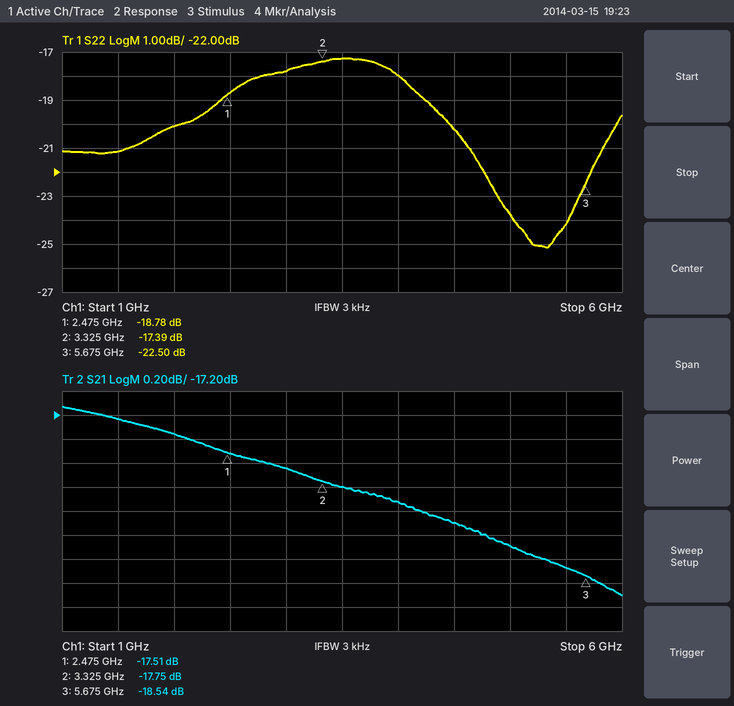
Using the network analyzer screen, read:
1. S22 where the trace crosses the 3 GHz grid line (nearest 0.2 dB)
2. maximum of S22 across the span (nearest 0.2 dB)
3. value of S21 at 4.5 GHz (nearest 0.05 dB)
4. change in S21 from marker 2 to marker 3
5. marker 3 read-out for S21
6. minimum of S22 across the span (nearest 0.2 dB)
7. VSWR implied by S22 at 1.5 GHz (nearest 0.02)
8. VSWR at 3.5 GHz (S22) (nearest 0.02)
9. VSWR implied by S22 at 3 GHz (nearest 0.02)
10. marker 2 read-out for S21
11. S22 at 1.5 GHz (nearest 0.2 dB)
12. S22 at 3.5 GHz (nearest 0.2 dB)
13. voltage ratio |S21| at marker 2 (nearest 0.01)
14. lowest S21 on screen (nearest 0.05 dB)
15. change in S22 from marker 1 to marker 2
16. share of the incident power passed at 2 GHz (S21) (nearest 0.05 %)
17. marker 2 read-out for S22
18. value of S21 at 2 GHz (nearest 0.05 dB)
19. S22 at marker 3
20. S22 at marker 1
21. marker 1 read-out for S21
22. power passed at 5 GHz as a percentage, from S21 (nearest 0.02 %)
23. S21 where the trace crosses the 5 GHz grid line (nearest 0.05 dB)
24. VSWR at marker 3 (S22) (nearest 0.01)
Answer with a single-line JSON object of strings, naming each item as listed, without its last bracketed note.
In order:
{"S22 where the trace crosses the 3 GHz grid line": "-17.8 dB", "maximum of S22 across the span": "-17.2 dB", "value of S21 at 4.5 GHz": "-18.10 dB", "change in S21 from marker 2 to marker 3": "-0.79 dB", "marker 3 read-out for S21": "-18.54 dB", "minimum of S22 across the span": "-25.2 dB", "VSWR implied by S22 at 1.5 GHz": "1.20", "VSWR at 3.5 GHz (S22)": "1.32", "VSWR implied by S22 at 3 GHz": "1.30", "marker 2 read-out for S21": "-17.75 dB", "S22 at 1.5 GHz": "-21.2 dB", "S22 at 3.5 GHz": "-17.2 dB", "voltage ratio |S21| at marker 2": "0.13", "lowest S21 on screen": "-18.70 dB", "change in S22 from marker 1 to marker 2": "1.39 dB", "share of the incident power passed at 2 GHz (S21)": "1.85 %", "marker 2 read-out for S22": "-17.39 dB", "value of S21 at 2 GHz": "-17.35 dB", "S22 at marker 3": "-22.50 dB", "S22 at marker 1": "-18.78 dB", "marker 1 read-out for S21": "-17.51 dB", "power passed at 5 GHz as a percentage, from S21": "1.48 %", "S21 where the trace crosses the 5 GHz grid line": "-18.30 dB", "VSWR at marker 3 (S22)": "1.16"}
